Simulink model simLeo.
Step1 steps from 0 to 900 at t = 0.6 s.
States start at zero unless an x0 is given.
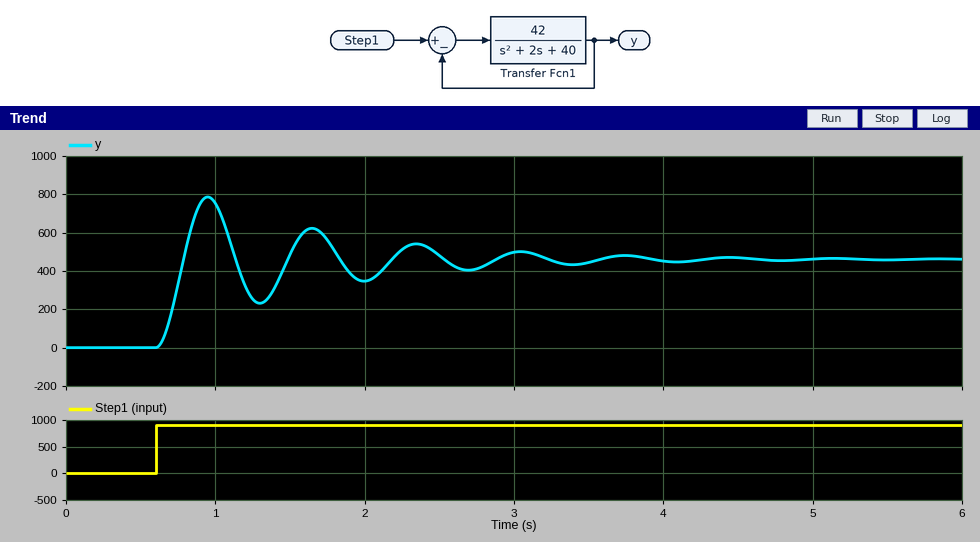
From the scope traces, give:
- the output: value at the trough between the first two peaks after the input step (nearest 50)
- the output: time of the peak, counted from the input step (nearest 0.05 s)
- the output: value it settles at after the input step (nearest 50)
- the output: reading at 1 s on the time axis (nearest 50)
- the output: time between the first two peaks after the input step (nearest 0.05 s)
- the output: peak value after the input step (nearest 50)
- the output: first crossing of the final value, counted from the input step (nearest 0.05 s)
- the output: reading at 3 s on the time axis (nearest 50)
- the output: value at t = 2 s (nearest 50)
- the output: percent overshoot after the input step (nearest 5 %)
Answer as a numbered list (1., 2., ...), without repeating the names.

1. 250
2. 0.35 s
3. 450
4. 750
5. 0.70 s
6. 800
7. 0.20 s
8. 500
9. 350
10. 70 %
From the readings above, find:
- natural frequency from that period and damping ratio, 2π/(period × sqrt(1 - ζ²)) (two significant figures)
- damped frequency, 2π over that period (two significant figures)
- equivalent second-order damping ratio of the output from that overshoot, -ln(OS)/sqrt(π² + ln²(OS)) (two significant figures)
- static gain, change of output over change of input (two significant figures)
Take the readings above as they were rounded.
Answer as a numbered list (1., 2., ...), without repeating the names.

1. 9.0 rad/s
2. 9.0 rad/s
3. 0.11
4. 0.50
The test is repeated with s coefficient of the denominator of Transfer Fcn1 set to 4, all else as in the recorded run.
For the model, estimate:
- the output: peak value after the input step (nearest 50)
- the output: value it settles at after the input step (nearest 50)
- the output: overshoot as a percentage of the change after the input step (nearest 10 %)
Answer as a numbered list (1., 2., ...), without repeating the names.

1. 700
2. 450
3. 50 %
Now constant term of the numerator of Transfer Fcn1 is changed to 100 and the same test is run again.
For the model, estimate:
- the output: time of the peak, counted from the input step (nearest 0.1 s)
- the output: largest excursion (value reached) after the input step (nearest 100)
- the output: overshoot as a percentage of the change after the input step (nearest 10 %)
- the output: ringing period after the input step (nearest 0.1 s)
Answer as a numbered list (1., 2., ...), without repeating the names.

1. 0.3 s
2. 1100
3. 80 %
4. 0.5 s
